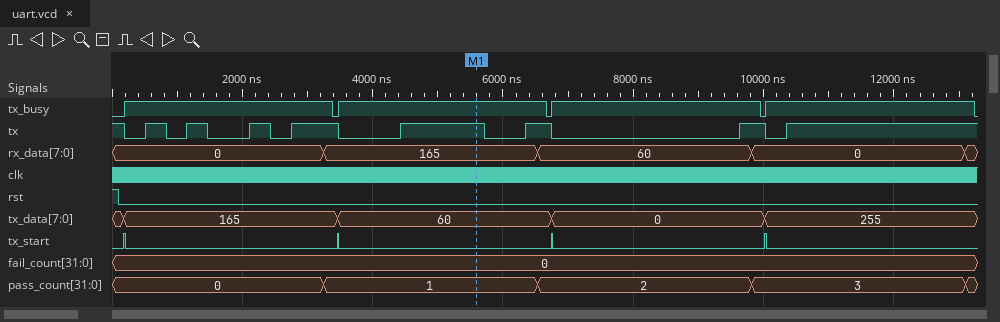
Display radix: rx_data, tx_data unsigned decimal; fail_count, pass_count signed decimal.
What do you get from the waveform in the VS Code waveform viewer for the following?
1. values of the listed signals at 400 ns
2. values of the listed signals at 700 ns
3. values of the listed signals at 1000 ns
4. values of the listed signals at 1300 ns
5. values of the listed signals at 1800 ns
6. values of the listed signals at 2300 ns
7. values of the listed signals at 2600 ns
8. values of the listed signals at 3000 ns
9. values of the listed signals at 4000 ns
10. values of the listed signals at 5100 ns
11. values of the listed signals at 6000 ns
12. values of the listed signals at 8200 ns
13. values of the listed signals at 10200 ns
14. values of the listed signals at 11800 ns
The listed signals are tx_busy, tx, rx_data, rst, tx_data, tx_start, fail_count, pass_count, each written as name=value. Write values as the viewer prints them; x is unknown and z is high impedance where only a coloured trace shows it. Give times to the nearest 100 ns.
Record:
tx_busy=1, tx=0, rx_data=0, rst=0, tx_data=165, tx_start=0, fail_count=0, pass_count=0
tx_busy=1, tx=1, rx_data=0, rst=0, tx_data=165, tx_start=0, fail_count=0, pass_count=0
tx_busy=1, tx=0, rx_data=0, rst=0, tx_data=165, tx_start=0, fail_count=0, pass_count=0
tx_busy=1, tx=1, rx_data=0, rst=0, tx_data=165, tx_start=0, fail_count=0, pass_count=0
tx_busy=1, tx=0, rx_data=0, rst=0, tx_data=165, tx_start=0, fail_count=0, pass_count=0
tx_busy=1, tx=1, rx_data=0, rst=0, tx_data=165, tx_start=0, fail_count=0, pass_count=0
tx_busy=1, tx=0, rx_data=0, rst=0, tx_data=165, tx_start=0, fail_count=0, pass_count=0
tx_busy=1, tx=1, rx_data=0, rst=0, tx_data=165, tx_start=0, fail_count=0, pass_count=0
tx_busy=1, tx=0, rx_data=165, rst=0, tx_data=60, tx_start=0, fail_count=0, pass_count=1
tx_busy=1, tx=1, rx_data=165, rst=0, tx_data=60, tx_start=0, fail_count=0, pass_count=1
tx_busy=1, tx=0, rx_data=165, rst=0, tx_data=60, tx_start=0, fail_count=0, pass_count=1
tx_busy=1, tx=0, rx_data=60, rst=0, tx_data=0, tx_start=0, fail_count=0, pass_count=2
tx_busy=1, tx=0, rx_data=0, rst=0, tx_data=255, tx_start=0, fail_count=0, pass_count=3
tx_busy=1, tx=1, rx_data=0, rst=0, tx_data=255, tx_start=0, fail_count=0, pass_count=3
